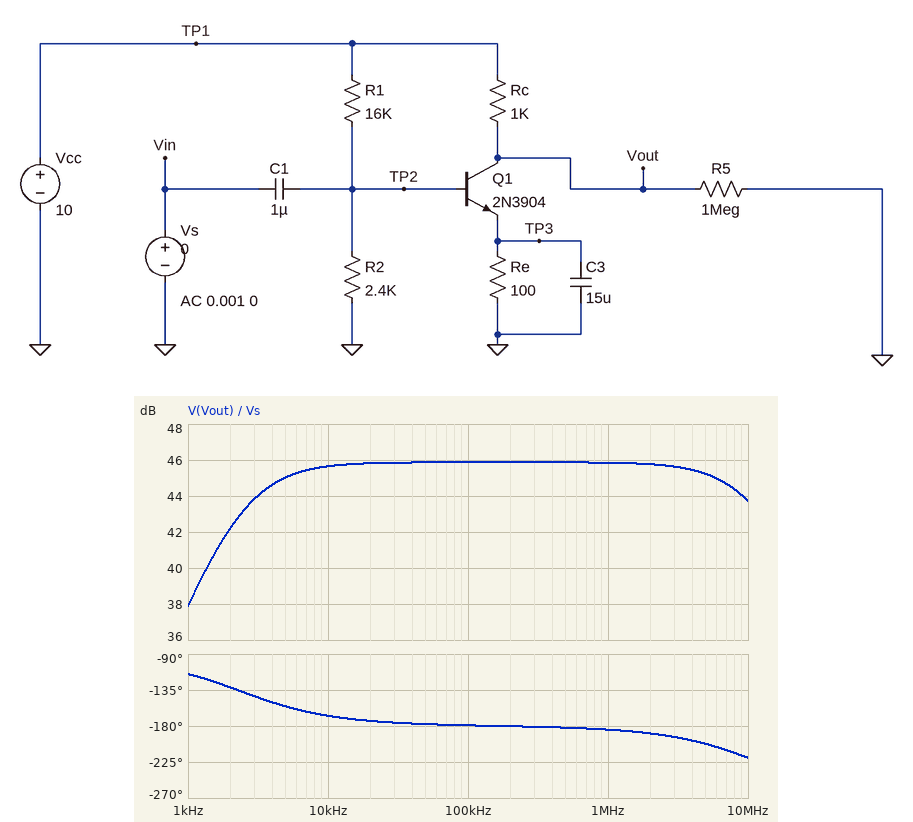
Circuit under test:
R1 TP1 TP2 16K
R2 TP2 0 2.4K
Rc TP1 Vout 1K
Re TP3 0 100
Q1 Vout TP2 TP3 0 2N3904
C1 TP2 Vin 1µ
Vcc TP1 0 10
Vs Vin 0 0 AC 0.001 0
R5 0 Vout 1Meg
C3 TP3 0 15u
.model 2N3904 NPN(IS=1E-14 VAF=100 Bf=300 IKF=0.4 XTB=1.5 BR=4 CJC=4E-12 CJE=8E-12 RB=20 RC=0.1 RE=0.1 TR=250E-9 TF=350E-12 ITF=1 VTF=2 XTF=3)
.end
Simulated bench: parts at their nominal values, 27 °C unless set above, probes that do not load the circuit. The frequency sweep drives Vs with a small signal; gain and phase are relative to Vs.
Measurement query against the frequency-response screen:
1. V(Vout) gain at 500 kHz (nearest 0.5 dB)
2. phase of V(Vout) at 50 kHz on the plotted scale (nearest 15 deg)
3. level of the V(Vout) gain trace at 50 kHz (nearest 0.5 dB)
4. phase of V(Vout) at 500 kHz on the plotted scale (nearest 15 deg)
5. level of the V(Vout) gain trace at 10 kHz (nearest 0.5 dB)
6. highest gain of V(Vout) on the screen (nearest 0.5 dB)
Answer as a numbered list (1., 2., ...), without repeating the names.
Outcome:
1. 46.0 dB
2. -180 deg
3. 46.0 dB
4. -180 deg
5. 45.5 dB
6. 46.0 dB
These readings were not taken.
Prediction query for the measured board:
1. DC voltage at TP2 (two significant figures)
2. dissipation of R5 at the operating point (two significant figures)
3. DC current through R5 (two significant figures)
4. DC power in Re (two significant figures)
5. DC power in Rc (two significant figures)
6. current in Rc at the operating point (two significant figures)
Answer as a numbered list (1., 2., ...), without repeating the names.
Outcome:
1. 1.3 V
2. 19 µW
3. 4.4 µA
4. 3.2 mW
5. 32 mW
6. 5.6 mA
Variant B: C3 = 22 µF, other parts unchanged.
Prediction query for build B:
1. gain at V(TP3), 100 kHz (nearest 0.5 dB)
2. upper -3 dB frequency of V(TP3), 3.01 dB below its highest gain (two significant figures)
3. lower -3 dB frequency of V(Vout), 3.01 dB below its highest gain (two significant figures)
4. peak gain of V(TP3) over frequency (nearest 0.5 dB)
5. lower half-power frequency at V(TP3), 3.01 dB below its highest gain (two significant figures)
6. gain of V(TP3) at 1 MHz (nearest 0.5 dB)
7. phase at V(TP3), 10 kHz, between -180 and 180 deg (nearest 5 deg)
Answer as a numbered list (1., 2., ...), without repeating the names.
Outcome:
1. -37.0 dB
2. 1.8 kHz
3. 1.6 kHz
4. -1.5 dB
5. 70 Hz
6. -57.0 dB
7. -80 deg
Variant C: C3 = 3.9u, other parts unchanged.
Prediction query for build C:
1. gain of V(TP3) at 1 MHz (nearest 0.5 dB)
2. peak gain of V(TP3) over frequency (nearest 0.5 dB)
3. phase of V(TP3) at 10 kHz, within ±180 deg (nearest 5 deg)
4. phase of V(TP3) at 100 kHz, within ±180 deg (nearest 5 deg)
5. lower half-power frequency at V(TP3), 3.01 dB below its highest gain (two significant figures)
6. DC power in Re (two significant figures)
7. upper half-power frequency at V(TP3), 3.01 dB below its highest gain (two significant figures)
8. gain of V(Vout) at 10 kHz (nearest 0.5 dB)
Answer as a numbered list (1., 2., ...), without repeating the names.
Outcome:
1. -42.0 dB
2. -0.5 dB
3. -50 deg
4. -85 deg
5. 79 Hz
6. 3.2 mW
7. 8.7 kHz
8. 43.5 dB
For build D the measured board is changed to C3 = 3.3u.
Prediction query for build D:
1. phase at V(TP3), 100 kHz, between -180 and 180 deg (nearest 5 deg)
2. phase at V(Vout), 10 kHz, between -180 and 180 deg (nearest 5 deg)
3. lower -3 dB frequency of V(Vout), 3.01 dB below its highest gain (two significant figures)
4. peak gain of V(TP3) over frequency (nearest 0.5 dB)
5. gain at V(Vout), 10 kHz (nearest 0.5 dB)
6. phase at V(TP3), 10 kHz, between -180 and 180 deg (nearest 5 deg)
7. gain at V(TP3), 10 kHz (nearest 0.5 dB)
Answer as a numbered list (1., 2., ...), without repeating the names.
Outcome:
1. -85 deg
2. -135 deg
3. 10 kHz
4. -0.5 dB
5. 43.0 dB
6. -45 deg
7. -3.5 dB
